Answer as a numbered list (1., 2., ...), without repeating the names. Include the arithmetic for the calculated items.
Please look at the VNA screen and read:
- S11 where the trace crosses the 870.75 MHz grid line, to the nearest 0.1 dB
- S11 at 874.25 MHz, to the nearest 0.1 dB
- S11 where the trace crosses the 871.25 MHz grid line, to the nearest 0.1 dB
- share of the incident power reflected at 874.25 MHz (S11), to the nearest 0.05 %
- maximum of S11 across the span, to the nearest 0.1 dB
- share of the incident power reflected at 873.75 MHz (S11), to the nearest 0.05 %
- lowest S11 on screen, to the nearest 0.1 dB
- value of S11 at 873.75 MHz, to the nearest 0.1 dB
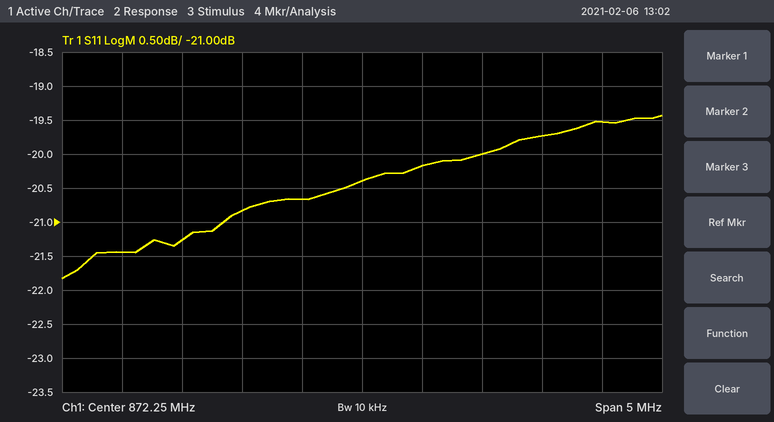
1. -21.3 dB
2. -19.5 dB
3. -20.8 dB
4. 10^(-19.5/10) ≈ 1.12 %, so 1.10 % to the nearest 0.05 %
5. -19.4 dB
6. 10^(-19.7/10) ≈ 1.07 %, so 1.05 % to the nearest 0.05 %
7. -21.8 dB
8. -19.7 dB
